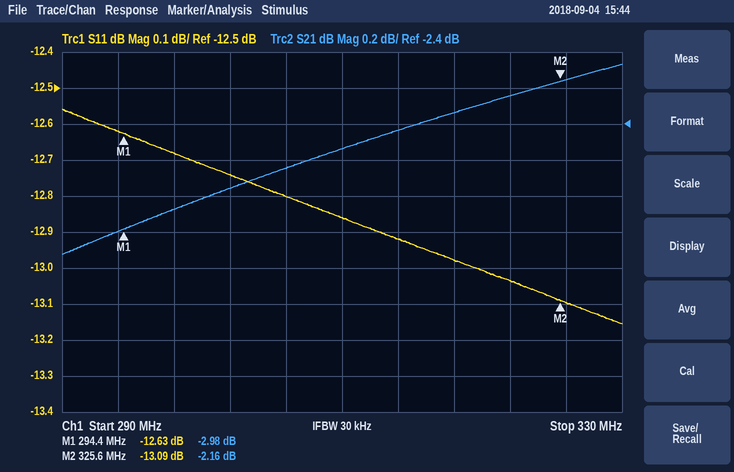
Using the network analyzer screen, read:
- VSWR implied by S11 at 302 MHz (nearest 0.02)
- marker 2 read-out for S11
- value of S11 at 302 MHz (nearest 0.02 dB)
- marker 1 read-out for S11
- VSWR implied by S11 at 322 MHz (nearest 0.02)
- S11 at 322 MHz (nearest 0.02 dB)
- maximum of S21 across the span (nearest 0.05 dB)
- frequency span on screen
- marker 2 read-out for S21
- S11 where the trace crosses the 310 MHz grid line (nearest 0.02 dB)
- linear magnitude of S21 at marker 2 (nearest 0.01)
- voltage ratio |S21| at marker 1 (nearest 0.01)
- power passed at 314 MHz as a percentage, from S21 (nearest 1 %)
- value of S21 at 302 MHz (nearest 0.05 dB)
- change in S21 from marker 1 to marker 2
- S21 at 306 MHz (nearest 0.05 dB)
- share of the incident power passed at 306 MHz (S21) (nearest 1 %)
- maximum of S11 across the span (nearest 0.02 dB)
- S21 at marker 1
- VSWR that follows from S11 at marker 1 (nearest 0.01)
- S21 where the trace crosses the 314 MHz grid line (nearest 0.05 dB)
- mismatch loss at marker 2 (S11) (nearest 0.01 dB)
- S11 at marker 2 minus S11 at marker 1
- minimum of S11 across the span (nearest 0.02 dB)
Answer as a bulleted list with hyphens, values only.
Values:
- 1.60
- -13.09 dB
- -12.74 dB
- -12.63 dB
- 1.58
- -13.04 dB
- -2.05 dB
- 40 MHz
- -2.16 dB
- -12.86 dB
- 0.78
- 0.71
- 57 %
- -2.75 dB
- 0.82 dB
- -2.65 dB
- 54 %
- -12.56 dB
- -2.98 dB
- 1.61
- -2.45 dB
- 0.22 dB
- -0.46 dB
- -13.16 dB
